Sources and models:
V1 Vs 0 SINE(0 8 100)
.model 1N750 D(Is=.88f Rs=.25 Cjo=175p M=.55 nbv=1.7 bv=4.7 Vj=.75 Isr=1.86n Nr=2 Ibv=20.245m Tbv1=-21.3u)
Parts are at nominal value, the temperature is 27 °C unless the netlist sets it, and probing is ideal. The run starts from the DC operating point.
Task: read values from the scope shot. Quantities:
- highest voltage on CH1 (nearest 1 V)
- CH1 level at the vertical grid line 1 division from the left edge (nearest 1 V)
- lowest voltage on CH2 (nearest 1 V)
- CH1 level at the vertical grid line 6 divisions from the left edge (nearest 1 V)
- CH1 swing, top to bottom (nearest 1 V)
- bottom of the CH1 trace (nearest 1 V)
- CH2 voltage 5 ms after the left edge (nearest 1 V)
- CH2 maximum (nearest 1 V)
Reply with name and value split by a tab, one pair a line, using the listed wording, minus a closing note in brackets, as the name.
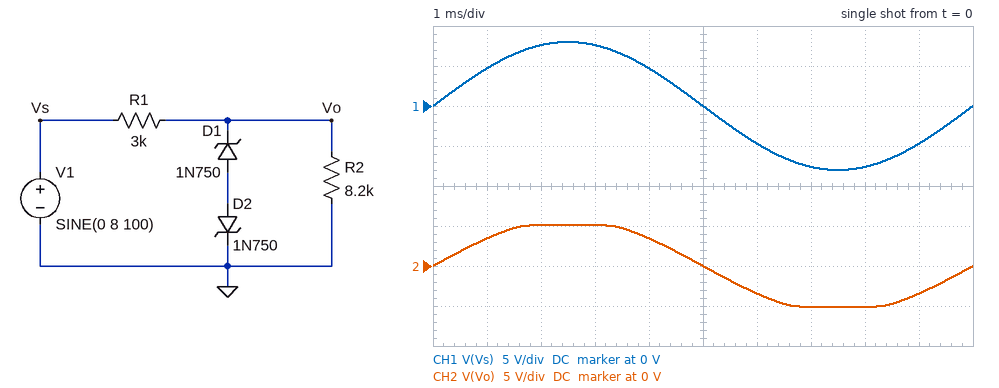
highest voltage on CH1	8 V
CH1 level at the vertical grid line 1 division from the left edge	5 V
lowest voltage on CH2	-5 V
CH1 level at the vertical grid line 6 divisions from the left edge	-5 V
CH1 swing, top to bottom	16 V
bottom of the CH1 trace	-8 V
CH2 voltage 5 ms after the left edge	0 V
CH2 maximum	5 V
